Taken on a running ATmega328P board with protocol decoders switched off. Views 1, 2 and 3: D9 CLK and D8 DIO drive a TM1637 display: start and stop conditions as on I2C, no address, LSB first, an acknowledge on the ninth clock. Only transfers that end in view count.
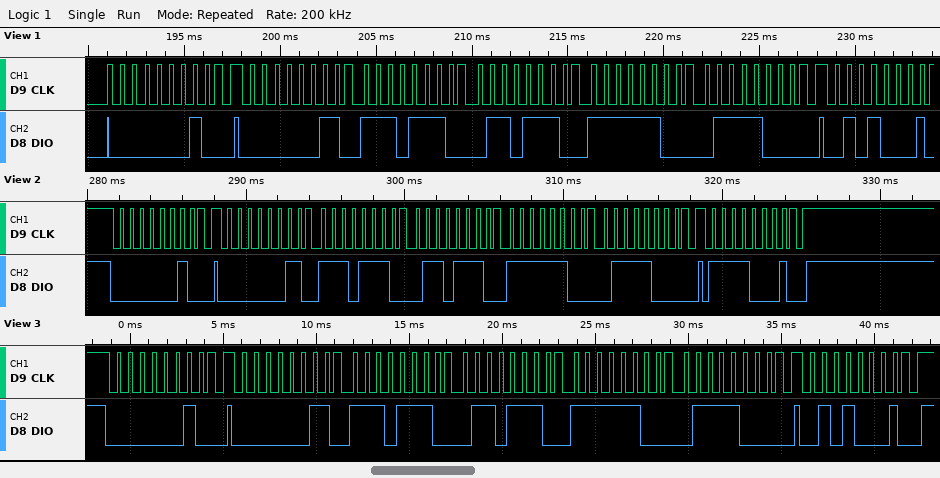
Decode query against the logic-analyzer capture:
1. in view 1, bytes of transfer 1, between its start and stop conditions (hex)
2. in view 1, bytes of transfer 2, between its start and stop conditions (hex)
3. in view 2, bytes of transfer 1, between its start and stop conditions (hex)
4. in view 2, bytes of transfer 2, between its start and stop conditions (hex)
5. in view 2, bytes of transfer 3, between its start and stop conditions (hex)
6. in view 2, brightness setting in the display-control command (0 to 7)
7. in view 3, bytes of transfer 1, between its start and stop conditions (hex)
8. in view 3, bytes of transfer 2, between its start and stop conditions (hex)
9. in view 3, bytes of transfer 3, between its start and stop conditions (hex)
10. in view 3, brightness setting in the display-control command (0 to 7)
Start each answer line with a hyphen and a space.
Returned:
- 40
- C0 77 76 3F 1E
- 40
- C0 77 76 3F 1E
- 8F
- 7
- 40
- C0 77 76 3F 1E
- 8A
- 2
